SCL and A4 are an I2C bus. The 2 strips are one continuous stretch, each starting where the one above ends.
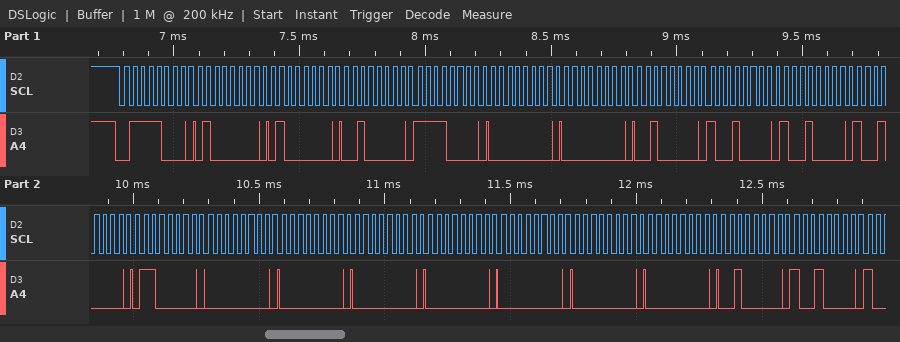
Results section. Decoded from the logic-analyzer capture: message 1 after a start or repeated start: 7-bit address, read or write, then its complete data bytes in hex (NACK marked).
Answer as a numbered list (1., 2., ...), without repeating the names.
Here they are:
1. 0x3C write: 40 40 20 F0 00 00 20 90 90 90 60 00 00 00 00 00 00 00 20 90
